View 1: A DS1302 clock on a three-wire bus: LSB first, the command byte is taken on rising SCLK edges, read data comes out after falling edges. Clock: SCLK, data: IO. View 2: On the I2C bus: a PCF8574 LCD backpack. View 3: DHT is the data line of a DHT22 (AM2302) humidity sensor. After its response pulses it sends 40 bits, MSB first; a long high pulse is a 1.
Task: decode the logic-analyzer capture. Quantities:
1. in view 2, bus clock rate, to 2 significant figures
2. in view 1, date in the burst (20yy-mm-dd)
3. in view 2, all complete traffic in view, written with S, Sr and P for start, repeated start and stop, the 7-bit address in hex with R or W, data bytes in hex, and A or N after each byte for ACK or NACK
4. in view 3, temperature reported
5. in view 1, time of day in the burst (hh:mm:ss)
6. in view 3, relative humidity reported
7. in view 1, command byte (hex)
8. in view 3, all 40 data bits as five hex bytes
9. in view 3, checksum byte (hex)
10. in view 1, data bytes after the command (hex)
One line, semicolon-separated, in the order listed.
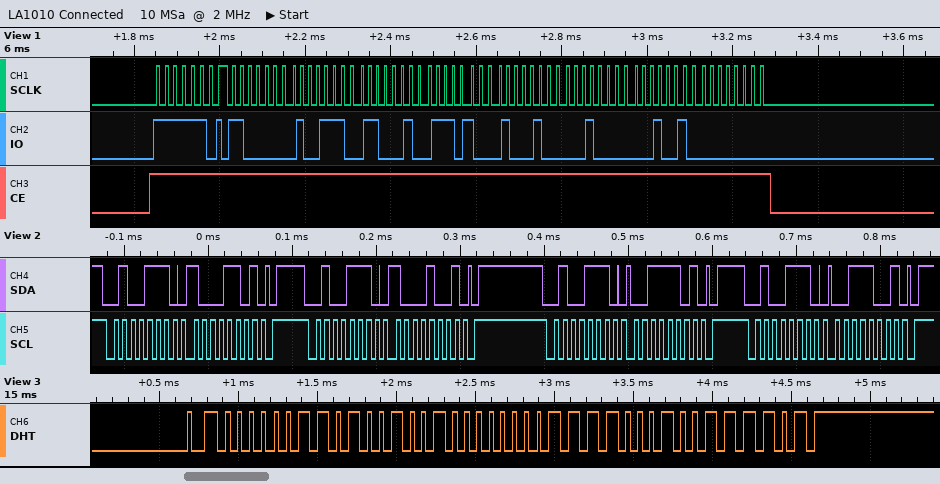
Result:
100 kHz; 2024-11-17; S 27W A 8D A P S 27W A 89 A P S 27W A 3D A P S 27W A 39 A P; 24.1 °C; 23:39:03; 84.1 %; 0xBF; 03 49 00 F1 3D; 0x3D; 03 39 23 17 11 04 24 00
